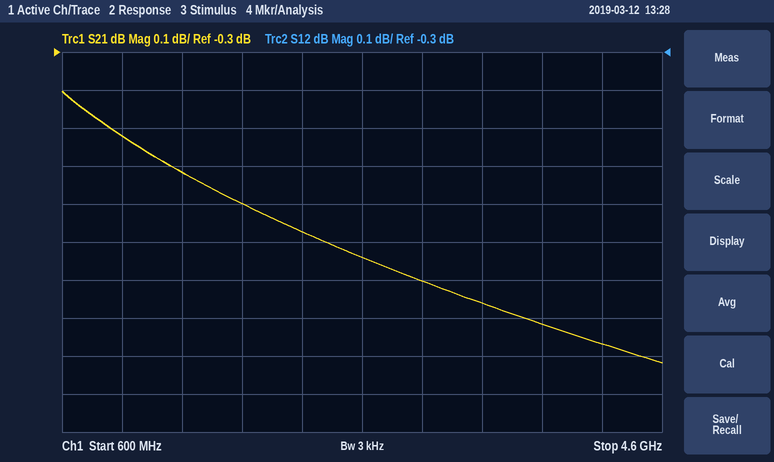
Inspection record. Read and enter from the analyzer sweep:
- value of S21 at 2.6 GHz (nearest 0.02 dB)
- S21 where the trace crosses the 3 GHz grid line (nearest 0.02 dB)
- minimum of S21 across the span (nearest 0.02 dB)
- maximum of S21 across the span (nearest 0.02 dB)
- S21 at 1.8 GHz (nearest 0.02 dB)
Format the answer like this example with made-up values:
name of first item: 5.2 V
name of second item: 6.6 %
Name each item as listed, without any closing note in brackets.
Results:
value of S21 at 2.6 GHz: -0.84 dB
S21 where the trace crosses the 3 GHz grid line: -0.90 dB
minimum of S21 across the span: -1.12 dB
maximum of S21 across the span: -0.40 dB
S21 at 1.8 GHz: -0.70 dB
